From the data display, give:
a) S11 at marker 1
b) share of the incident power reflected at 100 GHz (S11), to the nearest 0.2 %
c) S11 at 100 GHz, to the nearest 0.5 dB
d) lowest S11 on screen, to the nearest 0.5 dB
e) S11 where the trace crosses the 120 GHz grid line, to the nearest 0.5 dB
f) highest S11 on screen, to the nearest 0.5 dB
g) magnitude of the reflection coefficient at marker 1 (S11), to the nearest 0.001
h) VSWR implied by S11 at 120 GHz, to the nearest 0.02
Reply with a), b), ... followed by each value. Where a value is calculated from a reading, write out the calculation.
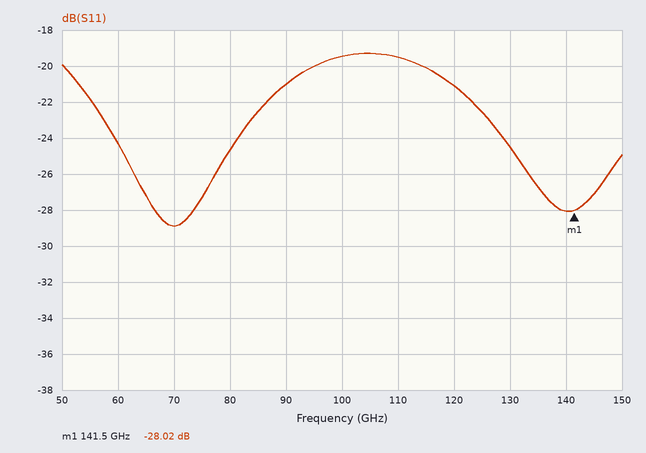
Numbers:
a) -28.02 dB
b) 10^(-19.5/10) ≈ 1.12 %, so 1.2 % to the nearest 0.2 %
c) -19.5 dB
d) -29.0 dB
e) -21.0 dB
f) -19.5 dB
g) 10^(-28.02/20) ≈ 0.040
h) |Γ| = 10^(-21/20) = 0.0891; VSWR = (1 + 0.0891)/(1 − 0.0891) ≈ 1.20
